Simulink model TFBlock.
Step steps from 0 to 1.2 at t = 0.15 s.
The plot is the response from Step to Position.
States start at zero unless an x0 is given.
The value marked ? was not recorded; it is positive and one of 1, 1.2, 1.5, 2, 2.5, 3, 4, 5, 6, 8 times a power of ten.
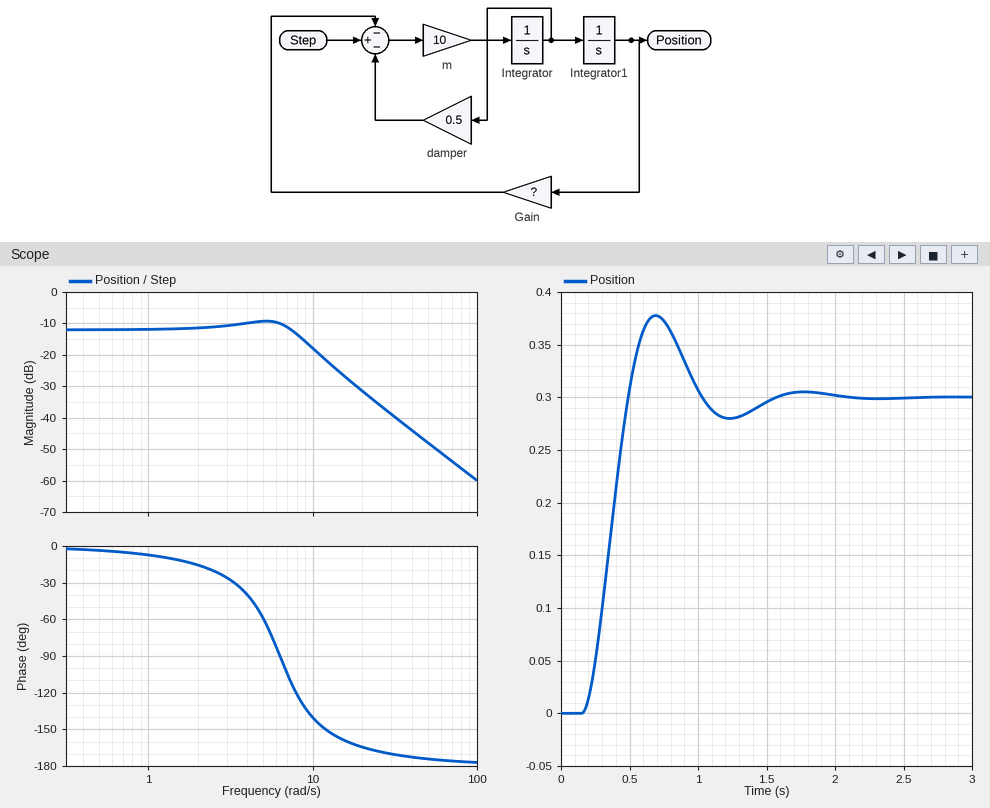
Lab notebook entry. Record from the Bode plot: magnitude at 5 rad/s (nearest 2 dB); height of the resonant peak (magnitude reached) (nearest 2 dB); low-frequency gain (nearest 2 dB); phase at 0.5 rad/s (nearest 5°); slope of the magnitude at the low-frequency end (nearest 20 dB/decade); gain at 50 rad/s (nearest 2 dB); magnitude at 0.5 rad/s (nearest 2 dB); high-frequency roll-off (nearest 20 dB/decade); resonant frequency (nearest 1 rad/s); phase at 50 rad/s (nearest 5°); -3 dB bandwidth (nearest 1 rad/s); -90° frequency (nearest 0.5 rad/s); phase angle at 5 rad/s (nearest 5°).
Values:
-10 dB
-10 dB
-12 dB
-5°
0 dB/decade
-48 dB
-12 dB
-40 dB/decade
5 rad/s
-175°
9 rad/s
6.5 rad/s
-60°
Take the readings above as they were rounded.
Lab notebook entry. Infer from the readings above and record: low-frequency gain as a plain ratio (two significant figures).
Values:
0.25
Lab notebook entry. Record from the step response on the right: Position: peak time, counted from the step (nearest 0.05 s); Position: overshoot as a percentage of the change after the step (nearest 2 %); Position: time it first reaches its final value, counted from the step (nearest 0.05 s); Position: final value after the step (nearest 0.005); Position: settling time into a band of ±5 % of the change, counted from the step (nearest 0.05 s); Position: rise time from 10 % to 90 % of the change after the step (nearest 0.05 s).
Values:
0.55 s
26 %
0.35 s
0.300
1.20 s
0.25 s
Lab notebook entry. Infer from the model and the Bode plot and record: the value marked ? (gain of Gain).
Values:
4
